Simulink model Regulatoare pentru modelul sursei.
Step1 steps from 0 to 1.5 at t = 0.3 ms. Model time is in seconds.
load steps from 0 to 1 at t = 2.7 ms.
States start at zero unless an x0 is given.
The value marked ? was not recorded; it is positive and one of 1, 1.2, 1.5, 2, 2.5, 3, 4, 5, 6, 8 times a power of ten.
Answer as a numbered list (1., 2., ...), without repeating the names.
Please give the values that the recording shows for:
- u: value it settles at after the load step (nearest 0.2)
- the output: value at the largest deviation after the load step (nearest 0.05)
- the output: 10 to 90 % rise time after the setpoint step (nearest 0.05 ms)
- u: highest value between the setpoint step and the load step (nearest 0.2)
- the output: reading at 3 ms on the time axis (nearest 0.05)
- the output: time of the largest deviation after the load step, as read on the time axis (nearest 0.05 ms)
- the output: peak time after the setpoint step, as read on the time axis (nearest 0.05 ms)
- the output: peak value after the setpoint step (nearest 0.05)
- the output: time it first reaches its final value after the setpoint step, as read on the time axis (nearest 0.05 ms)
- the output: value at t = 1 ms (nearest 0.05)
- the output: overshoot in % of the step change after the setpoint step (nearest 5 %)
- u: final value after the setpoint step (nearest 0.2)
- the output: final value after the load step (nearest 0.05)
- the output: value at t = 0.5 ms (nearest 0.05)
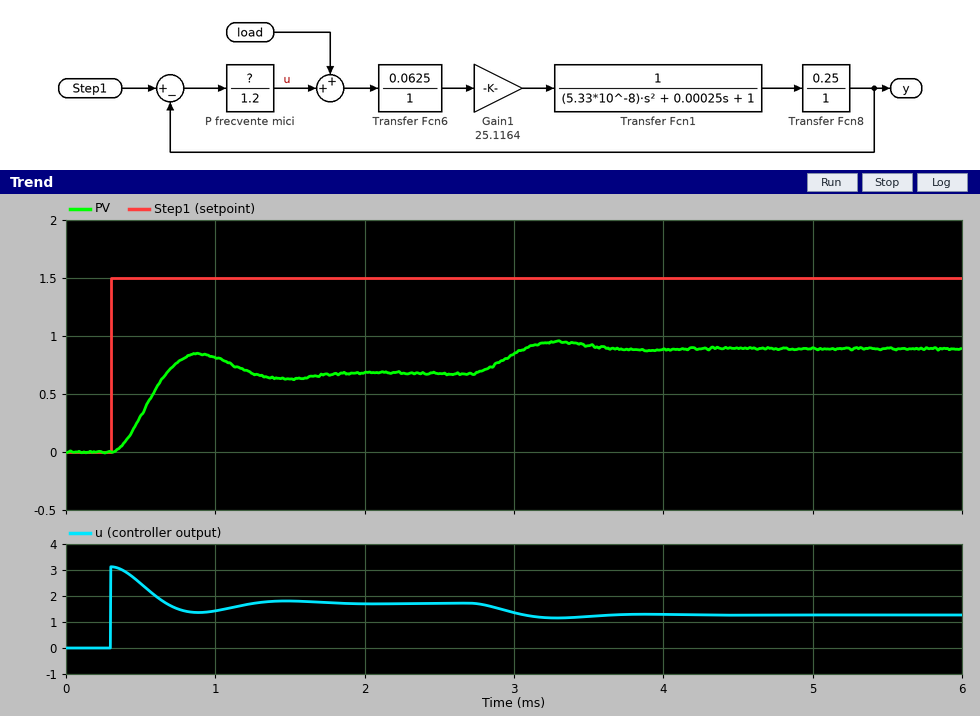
1. 1.2
2. 0.95
3. 0.25 ms
4. 3.2
5. 0.85
6. 3.30 ms
7. 0.90 ms
8. 0.85
9. 0.65 ms
10. 0.80
11. 25 %
12. 1.8
13. 0.90
14. 0.30
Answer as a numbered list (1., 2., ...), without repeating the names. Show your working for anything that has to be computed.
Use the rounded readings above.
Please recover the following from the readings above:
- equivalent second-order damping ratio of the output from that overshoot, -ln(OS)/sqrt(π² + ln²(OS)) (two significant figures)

1. ln(0.25) = -1.386; 1.386 / sqrt(9.870 + 1.922) = 0.40
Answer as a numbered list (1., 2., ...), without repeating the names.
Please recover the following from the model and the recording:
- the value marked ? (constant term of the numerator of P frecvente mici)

1. 2.5
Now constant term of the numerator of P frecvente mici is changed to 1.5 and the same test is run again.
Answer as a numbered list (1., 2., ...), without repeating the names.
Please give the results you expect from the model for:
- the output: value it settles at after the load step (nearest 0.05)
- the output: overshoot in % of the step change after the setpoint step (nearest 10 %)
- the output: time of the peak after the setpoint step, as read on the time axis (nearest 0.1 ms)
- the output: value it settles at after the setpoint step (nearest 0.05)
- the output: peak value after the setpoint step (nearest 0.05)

1. 0.75
2. 20 %
3. 1.0 ms
4. 0.50
5. 0.60
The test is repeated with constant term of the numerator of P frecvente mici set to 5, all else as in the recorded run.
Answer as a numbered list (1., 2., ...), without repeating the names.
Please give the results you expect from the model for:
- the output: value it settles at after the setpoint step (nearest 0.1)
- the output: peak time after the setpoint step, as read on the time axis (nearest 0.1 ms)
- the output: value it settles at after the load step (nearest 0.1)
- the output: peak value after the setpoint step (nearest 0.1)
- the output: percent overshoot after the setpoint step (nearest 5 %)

1. 0.9
2. 0.8 ms
3. 1.1
4. 1.2
5. 35 %
